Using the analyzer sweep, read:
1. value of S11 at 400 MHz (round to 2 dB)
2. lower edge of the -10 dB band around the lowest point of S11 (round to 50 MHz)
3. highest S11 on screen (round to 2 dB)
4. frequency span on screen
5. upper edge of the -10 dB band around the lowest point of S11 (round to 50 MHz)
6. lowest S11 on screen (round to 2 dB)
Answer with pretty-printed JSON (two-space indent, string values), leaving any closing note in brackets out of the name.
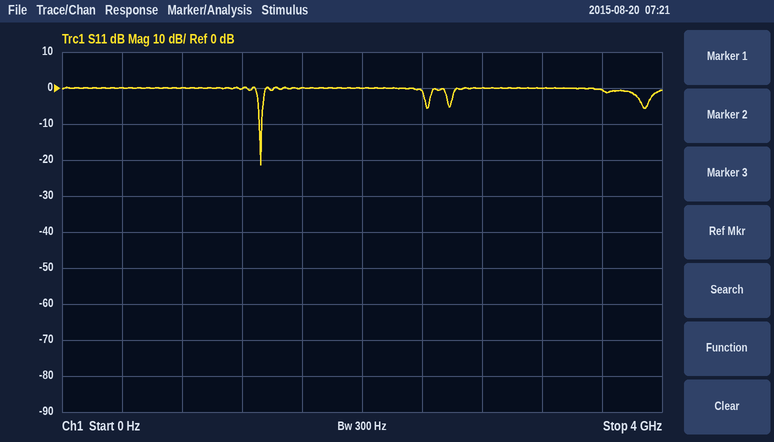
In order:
{
  "value of S11 at 400 MHz": "0 dB",
  "lower edge of the -10 dB band around the lowest point of S11": "1.30 GHz",
  "highest S11 on screen": "0 dB",
  "frequency span on screen": "4 GHz",
  "upper edge of the -10 dB band around the lowest point of S11": "1.35 GHz",
  "lowest S11 on screen": "-22 dB"
}
